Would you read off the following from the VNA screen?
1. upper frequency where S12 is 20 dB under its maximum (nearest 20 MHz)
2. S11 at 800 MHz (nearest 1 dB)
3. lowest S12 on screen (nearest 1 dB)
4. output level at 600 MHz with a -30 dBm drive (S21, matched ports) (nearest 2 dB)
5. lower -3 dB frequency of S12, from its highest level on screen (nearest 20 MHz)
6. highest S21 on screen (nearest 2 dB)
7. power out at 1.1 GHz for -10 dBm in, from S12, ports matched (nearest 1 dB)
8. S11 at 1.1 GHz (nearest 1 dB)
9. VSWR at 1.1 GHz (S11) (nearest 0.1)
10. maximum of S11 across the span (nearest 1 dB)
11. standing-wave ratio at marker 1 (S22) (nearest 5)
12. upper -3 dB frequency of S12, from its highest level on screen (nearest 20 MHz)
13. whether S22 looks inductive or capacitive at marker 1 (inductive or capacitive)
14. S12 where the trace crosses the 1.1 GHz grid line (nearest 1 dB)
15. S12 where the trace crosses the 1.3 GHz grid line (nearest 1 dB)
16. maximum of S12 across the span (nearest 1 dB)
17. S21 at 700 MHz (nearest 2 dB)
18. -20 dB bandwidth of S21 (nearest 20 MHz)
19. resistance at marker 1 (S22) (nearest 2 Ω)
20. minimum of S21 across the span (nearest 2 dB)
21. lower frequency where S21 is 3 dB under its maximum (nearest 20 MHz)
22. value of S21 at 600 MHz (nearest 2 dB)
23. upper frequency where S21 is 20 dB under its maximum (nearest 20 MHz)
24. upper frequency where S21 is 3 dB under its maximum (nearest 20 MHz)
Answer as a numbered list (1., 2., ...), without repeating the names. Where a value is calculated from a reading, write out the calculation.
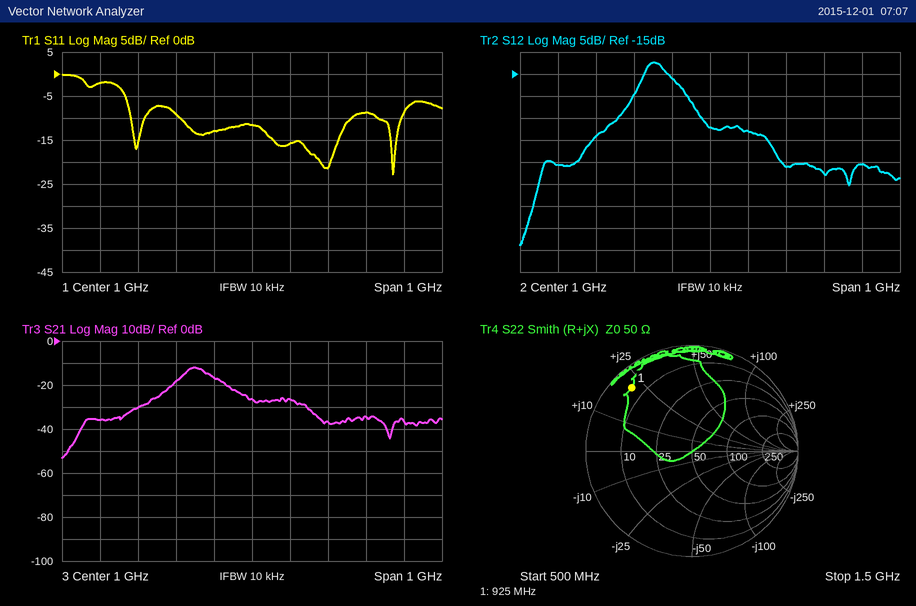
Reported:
1. 1.16 GHz
2. -9 dB
3. -54 dB
4. -30 dBm + (-36 dB) = -66 dBm
5. 820 MHz
6. -12 dB
7. -10 dBm + (-28 dB) = -38 dBm
8. -16 dB
9. |Γ| = 10^(-16/20) = 0.1585; VSWR = (1 + 0.1585)/(1 − 0.1585) ≈ 1.4
10. 0 dB
11. 10
12. 900 MHz
13. inductive
14. -28 dB
15. -38 dB
16. -12 dB
17. -30 dB
18. 1.16 GHz − 680 MHz = 480 MHz
19. 6 Ω
20. -54 dB
21. 820 MHz
22. -36 dB
23. 1.16 GHz
24. 880 MHz
